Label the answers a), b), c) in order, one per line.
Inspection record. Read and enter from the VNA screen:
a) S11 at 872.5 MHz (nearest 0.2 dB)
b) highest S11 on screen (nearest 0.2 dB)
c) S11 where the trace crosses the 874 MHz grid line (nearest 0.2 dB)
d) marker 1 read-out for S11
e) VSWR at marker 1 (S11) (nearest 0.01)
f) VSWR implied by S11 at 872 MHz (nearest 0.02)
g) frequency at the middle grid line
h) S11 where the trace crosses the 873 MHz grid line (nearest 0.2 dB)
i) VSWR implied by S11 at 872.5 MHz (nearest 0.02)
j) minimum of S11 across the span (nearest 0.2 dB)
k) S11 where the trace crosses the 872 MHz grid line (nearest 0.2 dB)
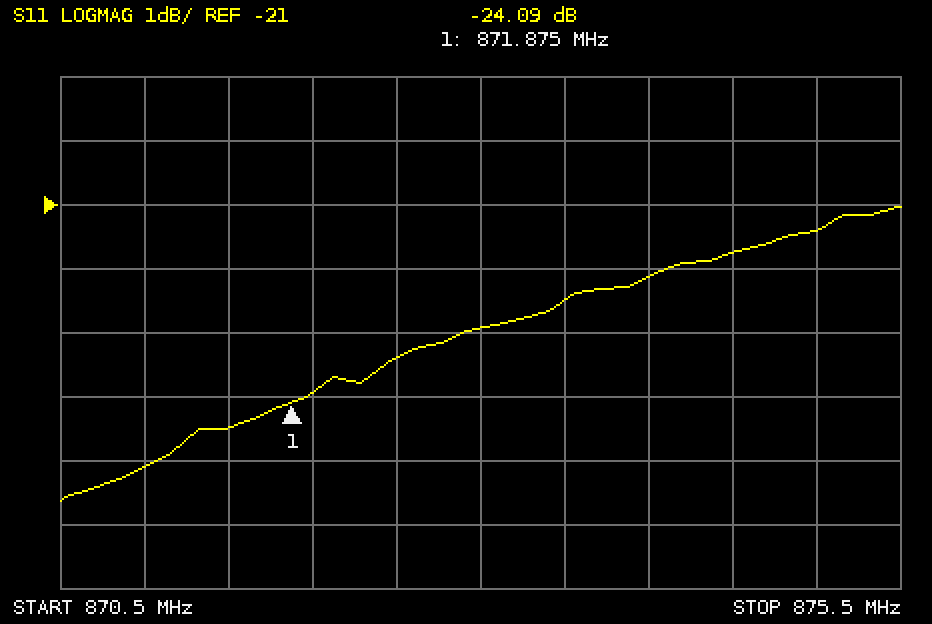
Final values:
a) -23.4 dB
b) -21.0 dB
c) -22.2 dB
d) -24.09 dB
e) 1.13
f) 1.14
g) 873 MHz
h) -23.0 dB
i) 1.14
j) -25.6 dB
k) -24.0 dB
